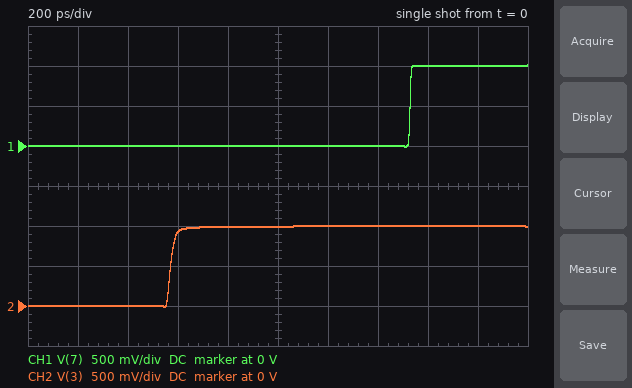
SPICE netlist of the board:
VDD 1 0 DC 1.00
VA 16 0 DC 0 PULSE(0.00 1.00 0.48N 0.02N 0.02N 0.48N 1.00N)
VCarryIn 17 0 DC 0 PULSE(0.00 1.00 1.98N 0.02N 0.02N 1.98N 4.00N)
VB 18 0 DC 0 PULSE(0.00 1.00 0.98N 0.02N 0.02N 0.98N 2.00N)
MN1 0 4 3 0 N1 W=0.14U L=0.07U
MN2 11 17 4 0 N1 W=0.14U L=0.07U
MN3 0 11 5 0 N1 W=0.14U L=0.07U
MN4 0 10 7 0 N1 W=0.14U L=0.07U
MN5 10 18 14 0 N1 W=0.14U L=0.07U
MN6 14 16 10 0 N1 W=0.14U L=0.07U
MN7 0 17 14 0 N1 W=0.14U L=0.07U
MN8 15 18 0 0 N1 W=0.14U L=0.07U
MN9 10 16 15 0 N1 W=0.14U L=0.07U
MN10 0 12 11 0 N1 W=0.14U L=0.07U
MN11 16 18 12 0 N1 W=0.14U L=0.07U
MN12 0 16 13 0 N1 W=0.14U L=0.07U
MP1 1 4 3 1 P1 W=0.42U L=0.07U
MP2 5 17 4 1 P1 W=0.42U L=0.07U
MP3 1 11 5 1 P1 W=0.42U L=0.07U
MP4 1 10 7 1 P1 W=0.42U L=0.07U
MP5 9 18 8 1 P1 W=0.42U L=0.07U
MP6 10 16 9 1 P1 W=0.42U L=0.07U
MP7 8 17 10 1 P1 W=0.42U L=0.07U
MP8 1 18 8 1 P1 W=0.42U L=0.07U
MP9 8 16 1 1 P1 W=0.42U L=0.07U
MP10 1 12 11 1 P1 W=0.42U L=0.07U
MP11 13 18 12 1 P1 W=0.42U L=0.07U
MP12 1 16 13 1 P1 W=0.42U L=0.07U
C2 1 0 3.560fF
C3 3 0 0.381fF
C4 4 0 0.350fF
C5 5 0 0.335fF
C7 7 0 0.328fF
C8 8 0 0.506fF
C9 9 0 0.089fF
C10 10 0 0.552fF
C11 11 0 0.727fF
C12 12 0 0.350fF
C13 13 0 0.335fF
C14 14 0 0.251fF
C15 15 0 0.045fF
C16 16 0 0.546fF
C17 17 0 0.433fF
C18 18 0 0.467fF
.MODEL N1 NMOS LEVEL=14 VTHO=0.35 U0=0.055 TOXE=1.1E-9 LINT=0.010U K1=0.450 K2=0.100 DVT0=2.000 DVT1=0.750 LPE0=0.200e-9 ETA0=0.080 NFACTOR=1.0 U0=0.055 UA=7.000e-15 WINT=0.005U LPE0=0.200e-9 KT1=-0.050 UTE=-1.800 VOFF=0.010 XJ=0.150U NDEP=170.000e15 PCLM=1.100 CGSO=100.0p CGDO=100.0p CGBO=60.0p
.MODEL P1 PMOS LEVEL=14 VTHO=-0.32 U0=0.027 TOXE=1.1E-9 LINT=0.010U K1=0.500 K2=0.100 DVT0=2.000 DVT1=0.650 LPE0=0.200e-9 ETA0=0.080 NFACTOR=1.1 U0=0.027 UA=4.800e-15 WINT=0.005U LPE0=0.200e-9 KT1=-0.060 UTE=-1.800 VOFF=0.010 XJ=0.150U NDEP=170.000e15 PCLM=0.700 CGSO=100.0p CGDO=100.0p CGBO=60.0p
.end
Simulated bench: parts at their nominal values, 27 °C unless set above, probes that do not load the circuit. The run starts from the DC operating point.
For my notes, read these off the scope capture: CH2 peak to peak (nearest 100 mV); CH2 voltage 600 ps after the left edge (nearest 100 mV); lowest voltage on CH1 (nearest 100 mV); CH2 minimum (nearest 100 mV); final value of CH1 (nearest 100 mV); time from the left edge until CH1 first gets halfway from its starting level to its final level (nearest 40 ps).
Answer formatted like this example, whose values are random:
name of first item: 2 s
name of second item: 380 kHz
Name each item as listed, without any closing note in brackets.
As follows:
CH2 peak to peak: 1.0 V
CH2 voltage 600 ps after the left edge: 900 mV
lowest voltage on CH1: 0 V
CH2 minimum: 0 V
final value of CH1: 1.0 V
time from the left edge until CH1 first gets halfway from its starting level to its final level: 1.52 ns
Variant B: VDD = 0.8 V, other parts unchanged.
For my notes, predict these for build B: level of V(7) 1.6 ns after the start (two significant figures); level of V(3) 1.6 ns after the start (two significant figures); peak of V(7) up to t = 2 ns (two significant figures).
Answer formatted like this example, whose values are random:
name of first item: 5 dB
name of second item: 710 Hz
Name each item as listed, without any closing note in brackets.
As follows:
level of V(7) 1.6 ns after the start: 800 mV
level of V(3) 1.6 ns after the start: 790 mV
peak of V(7) up to t = 2 ns: 810 mV
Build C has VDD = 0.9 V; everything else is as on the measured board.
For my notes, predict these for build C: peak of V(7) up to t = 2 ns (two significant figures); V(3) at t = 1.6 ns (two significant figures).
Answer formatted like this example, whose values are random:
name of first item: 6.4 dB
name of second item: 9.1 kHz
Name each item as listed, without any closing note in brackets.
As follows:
peak of V(7) up to t = 2 ns: 910 mV
V(3) at t = 1.6 ns: 900 mV
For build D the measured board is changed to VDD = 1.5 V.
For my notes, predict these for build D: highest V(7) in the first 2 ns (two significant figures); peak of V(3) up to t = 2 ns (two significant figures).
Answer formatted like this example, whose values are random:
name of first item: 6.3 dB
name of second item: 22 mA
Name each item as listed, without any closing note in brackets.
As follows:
highest V(7) in the first 2 ns: 140 mV
peak of V(3) up to t = 2 ns: 1.5 V
